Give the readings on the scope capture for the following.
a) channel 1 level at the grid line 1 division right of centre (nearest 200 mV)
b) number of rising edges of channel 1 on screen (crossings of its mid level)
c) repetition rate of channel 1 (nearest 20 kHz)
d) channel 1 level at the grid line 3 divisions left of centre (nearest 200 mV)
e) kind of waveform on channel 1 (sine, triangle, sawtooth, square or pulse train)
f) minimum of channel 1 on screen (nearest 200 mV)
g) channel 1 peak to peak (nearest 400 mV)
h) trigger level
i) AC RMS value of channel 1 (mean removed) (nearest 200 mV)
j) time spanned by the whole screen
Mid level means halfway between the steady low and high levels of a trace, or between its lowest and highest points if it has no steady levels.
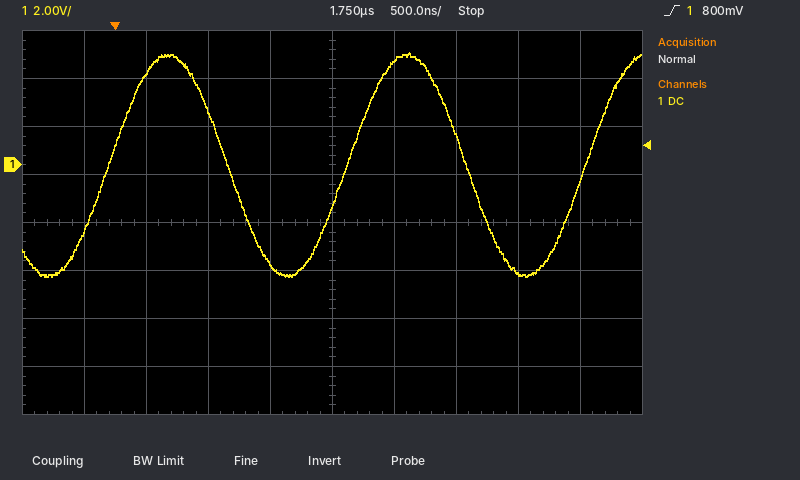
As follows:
4.4 V
3
520 kHz
3.8 V
sine
-4.6 V
9.2 V
800 mV
3.2 V
5 µs
